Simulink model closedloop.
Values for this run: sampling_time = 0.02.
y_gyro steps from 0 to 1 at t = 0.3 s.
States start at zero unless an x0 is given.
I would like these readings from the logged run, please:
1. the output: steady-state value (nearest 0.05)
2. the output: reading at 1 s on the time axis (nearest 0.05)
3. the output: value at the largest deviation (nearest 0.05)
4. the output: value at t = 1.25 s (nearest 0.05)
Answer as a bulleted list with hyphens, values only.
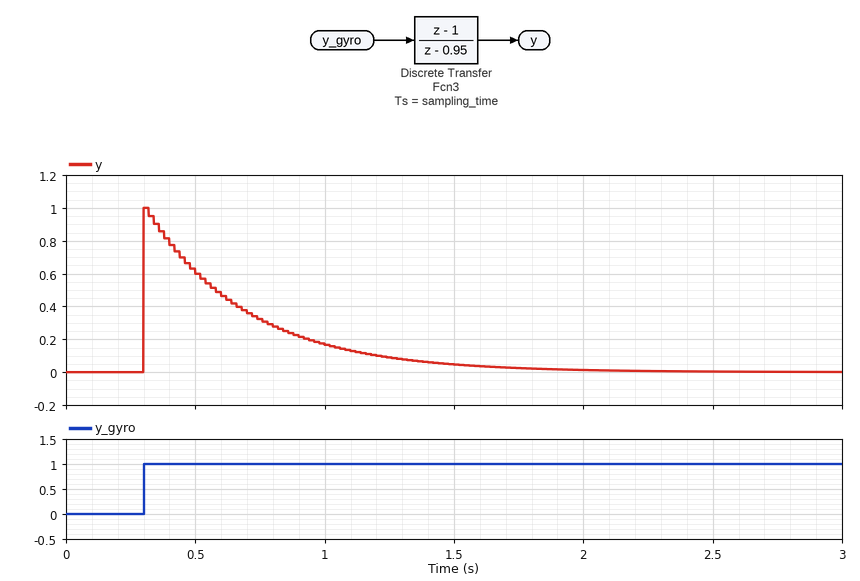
- 0.00
- 0.15
- 1.00
- 0.10
